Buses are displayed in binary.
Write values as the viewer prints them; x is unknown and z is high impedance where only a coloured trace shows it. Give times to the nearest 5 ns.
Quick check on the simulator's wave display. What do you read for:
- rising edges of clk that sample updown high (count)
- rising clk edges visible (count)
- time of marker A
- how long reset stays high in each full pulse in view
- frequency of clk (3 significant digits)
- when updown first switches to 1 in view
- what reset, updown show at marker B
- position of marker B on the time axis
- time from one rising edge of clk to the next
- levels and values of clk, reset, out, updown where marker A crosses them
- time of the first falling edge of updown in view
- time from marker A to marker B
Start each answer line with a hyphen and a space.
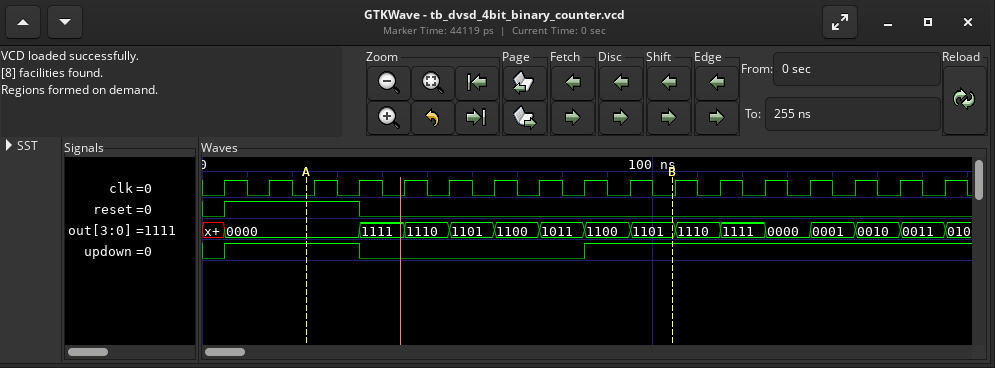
- 11
- 17
- 25 ns
- 30 ns
- 100 MHz
- 5 ns
- reset=0, updown=1
- 105 ns
- 10 ns
- clk=0, reset=1, out=0000, updown=1
- 35 ns
- 80 ns
